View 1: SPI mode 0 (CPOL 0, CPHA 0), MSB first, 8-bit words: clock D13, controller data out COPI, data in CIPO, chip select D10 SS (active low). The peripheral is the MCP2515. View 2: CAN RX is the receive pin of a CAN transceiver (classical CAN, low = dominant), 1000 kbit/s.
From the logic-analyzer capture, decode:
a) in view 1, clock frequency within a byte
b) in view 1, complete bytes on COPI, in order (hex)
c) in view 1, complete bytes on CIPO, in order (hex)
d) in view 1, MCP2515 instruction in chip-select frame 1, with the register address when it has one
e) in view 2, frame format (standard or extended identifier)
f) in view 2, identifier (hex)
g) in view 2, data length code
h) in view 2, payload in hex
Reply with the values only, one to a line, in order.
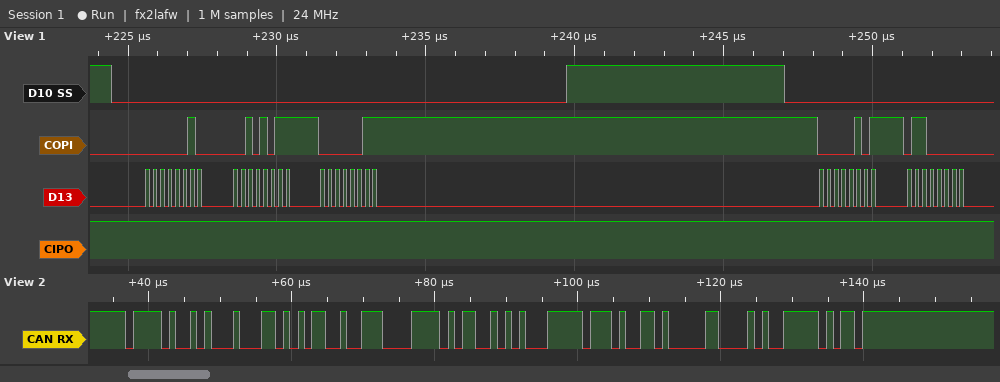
4 MHz
02 2B 03 05 60
FF FF FF FF FF
WRITE 0x2B
standard
0x7A5
8
D5 93 87 AC A8 FF 4D 04
